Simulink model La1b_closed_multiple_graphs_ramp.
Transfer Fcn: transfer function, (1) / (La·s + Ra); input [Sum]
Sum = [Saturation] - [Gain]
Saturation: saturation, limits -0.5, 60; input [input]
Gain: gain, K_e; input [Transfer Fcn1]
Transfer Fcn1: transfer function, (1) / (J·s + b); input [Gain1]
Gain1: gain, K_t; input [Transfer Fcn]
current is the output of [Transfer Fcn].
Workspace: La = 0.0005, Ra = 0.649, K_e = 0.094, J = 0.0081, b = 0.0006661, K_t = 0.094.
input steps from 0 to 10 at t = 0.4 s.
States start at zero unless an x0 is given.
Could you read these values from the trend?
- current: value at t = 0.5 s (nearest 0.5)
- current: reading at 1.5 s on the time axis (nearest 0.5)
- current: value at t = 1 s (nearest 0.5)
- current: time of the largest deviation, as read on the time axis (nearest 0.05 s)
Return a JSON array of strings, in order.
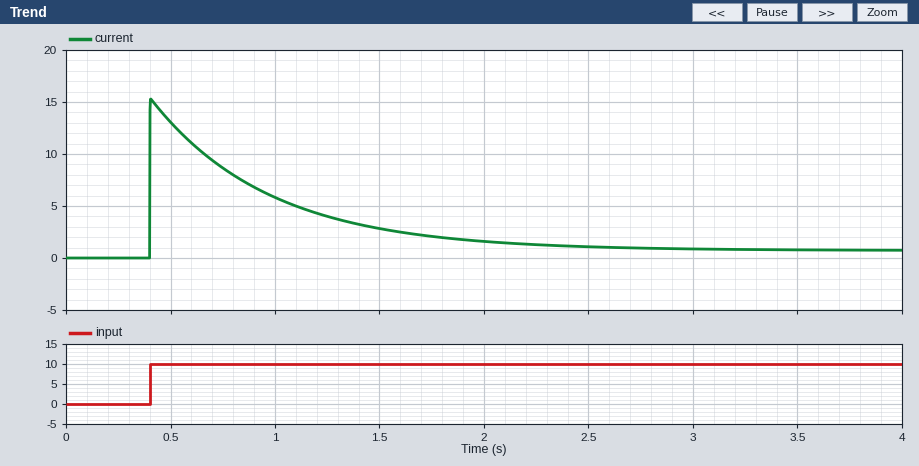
["13.0", "3.0", "6.0", "0.40 s"]
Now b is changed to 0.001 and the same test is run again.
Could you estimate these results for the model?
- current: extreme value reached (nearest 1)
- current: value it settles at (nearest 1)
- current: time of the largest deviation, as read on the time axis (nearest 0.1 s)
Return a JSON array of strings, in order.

["15", "1", "0.4 s"]
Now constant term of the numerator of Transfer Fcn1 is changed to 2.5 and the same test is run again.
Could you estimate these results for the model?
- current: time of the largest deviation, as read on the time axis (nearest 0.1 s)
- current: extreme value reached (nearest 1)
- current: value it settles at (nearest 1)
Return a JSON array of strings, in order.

["0.4 s", "15", "0"]
